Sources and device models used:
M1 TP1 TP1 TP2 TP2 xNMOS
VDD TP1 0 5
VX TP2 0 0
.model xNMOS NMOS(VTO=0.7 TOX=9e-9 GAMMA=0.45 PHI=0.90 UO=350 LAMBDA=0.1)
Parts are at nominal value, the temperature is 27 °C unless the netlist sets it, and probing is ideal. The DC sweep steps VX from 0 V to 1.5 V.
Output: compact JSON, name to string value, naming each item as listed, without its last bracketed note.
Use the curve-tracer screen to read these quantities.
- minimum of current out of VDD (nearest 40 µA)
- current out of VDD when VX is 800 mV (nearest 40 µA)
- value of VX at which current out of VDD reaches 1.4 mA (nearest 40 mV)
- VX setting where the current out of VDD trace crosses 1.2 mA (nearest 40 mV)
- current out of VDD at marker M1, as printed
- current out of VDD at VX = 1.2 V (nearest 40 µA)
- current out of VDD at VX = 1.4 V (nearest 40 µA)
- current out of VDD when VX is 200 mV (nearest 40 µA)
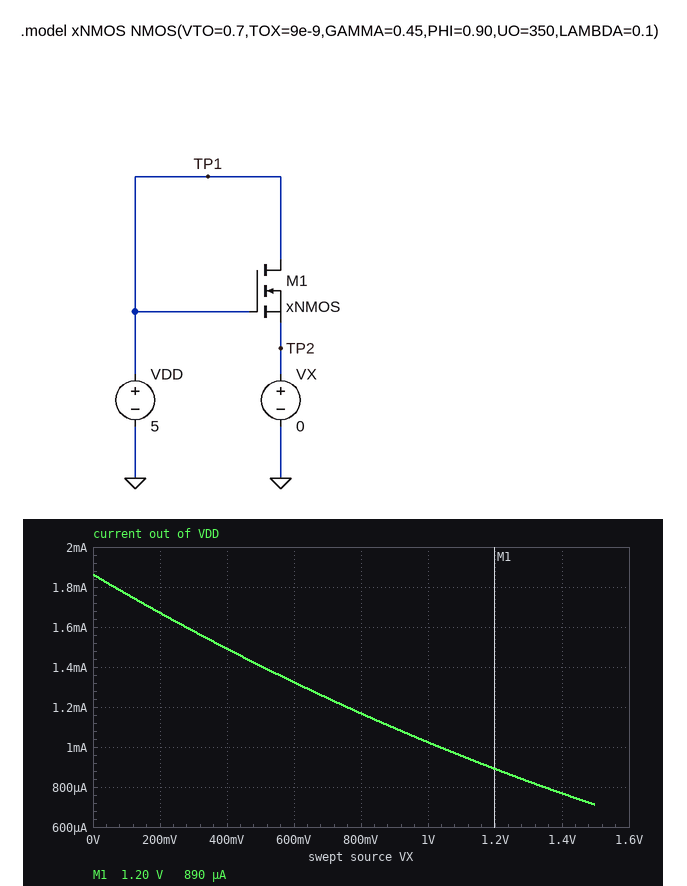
{"minimum of current out of VDD": "720 µA", "current out of VDD when VX is 800 mV": "1.16 mA", "value of VX at which current out of VDD reaches 1.4 mA": "520 mV", "VX setting where the current out of VDD trace crosses 1.2 mA": "760 mV", "current out of VDD at marker M1, as printed": "890 µA", "current out of VDD at VX = 1.2 V": "880 µA", "current out of VDD at VX = 1.4 V": "760 µA", "current out of VDD when VX is 200 mV": "1.68 mA"}
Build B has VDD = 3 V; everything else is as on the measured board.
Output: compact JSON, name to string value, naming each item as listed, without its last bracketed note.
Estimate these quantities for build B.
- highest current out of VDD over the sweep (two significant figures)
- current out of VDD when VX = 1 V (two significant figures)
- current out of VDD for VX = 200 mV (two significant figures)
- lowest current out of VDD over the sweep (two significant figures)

{"highest current out of VDD over the sweep": "460 µA", "current out of VDD when VX = 1 V": "140 µA", "current out of VDD for VX = 200 mV": "380 µA", "lowest current out of VDD over the sweep": "49 µA"}
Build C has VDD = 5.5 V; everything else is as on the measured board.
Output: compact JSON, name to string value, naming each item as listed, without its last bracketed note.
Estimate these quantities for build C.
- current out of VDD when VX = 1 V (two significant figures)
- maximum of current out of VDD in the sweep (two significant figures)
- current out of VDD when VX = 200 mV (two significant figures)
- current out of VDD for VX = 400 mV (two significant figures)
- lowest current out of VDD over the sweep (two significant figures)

{"current out of VDD when VX = 1 V": "1.4 mA", "maximum of current out of VDD in the sweep": "2.4 mA", "current out of VDD when VX = 200 mV": "2.2 mA", "current out of VDD for VX = 400 mV": "2.0 mA", "lowest current out of VDD over the sweep": "1.0 mA"}
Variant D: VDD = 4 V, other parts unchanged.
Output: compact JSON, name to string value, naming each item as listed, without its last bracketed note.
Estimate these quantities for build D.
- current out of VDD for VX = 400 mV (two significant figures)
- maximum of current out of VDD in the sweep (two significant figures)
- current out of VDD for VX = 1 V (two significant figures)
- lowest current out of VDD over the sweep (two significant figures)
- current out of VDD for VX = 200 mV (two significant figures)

{"current out of VDD for VX = 400 mV": "770 µA", "maximum of current out of VDD in the sweep": "1.0 mA", "current out of VDD for VX = 1 V": "460 µA", "lowest current out of VDD over the sweep": "270 µA", "current out of VDD for VX = 200 mV": "890 µA"}
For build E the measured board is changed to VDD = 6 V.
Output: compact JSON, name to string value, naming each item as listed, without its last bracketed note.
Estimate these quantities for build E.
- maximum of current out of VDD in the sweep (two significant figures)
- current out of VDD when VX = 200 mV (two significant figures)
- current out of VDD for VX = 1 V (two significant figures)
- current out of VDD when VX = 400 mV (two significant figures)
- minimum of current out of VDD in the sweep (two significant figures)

{"maximum of current out of VDD in the sweep": "3.0 mA", "current out of VDD when VX = 200 mV": "2.8 mA", "current out of VDD for VX = 1 V": "1.9 mA", "current out of VDD when VX = 400 mV": "2.5 mA", "minimum of current out of VDD in the sweep": "1.4 mA"}
